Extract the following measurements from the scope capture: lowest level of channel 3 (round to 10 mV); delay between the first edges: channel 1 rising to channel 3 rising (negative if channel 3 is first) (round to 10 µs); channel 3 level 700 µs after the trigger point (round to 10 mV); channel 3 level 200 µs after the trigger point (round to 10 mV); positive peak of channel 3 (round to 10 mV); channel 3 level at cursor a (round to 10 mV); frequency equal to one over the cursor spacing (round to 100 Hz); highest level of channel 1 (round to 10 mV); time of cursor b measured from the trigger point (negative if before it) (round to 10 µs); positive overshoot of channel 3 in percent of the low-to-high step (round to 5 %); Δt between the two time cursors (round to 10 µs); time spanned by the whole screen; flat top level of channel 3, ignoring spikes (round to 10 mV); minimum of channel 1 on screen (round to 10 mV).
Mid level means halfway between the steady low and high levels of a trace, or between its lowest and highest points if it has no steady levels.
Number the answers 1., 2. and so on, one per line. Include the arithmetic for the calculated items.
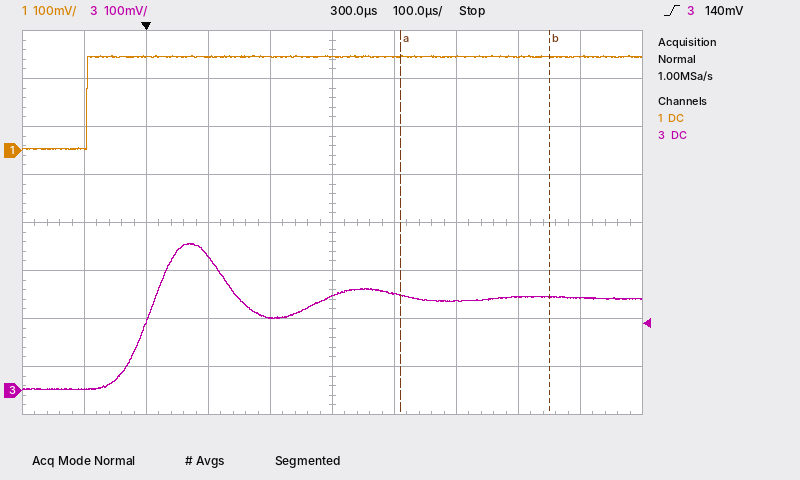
1. 0 mV
2. +80 µs
3. 190 mV
4. 150 mV
5. 310 mV
6. 200 mV
7. 1 / 240 µs ≈ 4.2 kHz
8. 200 mV
9. +650 µs
10. 60 %
11. 240 µs
12. 1 ms
13. 190 mV
14. 0 mV
